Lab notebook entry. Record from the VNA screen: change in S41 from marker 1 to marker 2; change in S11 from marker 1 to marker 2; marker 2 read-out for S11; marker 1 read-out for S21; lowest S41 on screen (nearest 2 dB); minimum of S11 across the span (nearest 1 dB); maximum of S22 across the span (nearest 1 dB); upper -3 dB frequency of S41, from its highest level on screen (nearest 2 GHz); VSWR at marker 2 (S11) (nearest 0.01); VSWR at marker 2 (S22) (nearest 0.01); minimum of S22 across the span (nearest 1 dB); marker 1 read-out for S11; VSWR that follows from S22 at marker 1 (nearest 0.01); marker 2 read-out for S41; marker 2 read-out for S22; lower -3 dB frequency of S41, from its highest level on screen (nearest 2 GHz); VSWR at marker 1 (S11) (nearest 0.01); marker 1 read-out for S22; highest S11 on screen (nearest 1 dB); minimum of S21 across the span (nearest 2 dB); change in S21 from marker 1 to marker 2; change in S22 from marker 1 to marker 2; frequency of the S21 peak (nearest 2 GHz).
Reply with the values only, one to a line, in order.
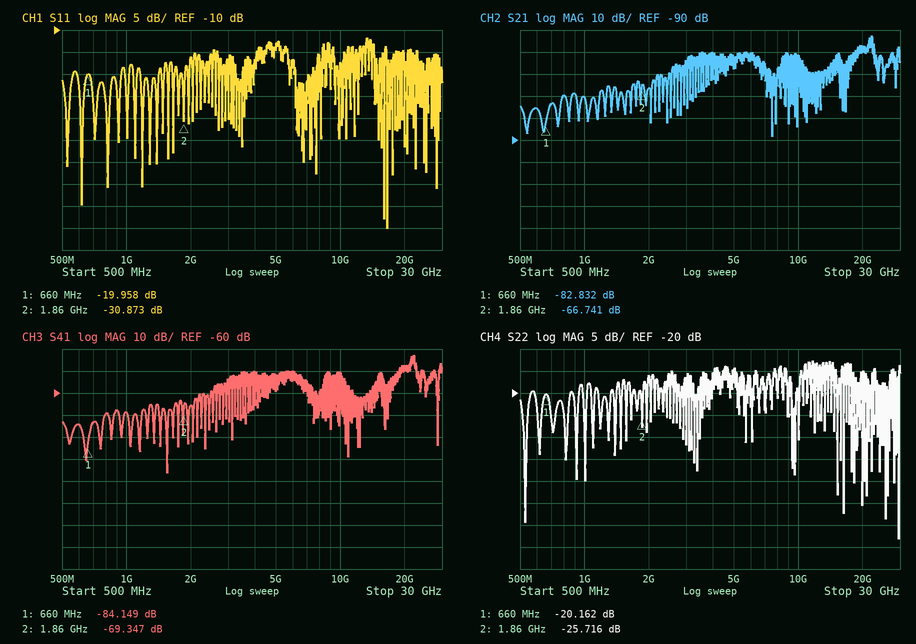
14.802 dB
-10.915 dB
-30.873 dB
-82.832 dB
-96 dB
-55 dB
-13 dB
22 GHz
1.06
1.11
-53 dB
-19.958 dB
1.22
-69.347 dB
-25.716 dB
22 GHz
1.22
-20.162 dB
-12 dB
-88 dB
16.091 dB
-5.554 dB
22 GHz
